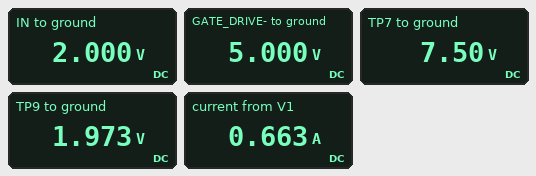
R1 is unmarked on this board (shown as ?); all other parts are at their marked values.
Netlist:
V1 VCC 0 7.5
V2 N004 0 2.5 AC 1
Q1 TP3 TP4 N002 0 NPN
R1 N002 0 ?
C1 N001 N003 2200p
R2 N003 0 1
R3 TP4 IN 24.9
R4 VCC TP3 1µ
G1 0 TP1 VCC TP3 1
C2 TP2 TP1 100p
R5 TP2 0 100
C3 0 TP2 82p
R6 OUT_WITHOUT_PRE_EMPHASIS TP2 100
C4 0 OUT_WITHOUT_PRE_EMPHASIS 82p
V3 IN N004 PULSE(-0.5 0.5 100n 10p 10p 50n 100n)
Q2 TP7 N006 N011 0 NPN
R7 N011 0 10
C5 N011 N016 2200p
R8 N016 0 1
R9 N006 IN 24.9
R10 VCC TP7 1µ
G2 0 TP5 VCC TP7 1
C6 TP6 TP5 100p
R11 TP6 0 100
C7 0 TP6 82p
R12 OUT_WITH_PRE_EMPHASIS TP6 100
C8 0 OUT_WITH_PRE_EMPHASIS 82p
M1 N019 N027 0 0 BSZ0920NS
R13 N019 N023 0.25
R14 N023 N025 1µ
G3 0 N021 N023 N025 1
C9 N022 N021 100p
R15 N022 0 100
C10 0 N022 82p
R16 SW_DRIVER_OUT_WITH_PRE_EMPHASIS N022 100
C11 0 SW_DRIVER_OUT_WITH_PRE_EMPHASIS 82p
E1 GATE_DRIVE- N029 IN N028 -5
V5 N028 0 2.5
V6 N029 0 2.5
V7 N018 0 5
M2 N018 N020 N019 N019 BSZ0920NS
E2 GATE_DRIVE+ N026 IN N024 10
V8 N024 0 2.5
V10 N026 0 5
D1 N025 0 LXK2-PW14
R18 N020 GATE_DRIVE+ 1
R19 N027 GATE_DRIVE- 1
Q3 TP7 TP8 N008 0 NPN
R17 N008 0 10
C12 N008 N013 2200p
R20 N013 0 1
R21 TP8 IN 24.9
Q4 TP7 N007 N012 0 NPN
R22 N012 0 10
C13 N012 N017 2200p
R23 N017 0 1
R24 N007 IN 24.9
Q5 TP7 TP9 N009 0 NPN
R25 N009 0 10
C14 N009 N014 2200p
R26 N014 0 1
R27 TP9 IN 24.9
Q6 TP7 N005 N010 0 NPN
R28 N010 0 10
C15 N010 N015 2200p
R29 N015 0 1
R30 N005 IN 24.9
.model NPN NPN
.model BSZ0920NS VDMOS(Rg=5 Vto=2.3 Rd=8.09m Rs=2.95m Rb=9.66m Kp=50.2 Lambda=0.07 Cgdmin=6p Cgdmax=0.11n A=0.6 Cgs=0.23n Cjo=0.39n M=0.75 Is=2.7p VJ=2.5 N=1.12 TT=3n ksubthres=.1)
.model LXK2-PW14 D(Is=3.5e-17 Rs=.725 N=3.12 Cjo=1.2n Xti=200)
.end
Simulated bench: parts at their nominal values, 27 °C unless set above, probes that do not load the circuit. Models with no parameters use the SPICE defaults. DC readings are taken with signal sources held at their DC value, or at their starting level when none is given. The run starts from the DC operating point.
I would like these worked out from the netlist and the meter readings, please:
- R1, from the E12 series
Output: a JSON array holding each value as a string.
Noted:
["8.2 Ω"]
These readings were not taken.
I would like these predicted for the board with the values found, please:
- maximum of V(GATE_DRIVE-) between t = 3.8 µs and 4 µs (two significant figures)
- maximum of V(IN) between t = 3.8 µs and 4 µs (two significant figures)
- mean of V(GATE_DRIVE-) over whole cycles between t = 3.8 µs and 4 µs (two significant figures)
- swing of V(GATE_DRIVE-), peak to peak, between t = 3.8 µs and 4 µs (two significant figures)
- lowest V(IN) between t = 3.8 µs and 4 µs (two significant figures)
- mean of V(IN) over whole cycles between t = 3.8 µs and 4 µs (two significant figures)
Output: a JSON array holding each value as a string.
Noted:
["5.0 V", "3.0 V", "2.5 V", "5.0 V", "2.0 V", "2.5 V"]
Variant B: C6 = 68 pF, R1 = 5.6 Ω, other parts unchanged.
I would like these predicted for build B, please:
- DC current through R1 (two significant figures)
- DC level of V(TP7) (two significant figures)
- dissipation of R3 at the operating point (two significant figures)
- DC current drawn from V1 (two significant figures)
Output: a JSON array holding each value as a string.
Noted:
["190 mA", "7.5 V", "85 µW", "720 mA"]
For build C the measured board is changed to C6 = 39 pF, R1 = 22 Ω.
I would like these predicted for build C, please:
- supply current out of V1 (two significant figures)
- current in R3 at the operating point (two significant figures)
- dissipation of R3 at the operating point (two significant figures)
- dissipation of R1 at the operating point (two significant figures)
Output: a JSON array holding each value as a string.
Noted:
["580 mA", "500 µA", "6.2 µW", "56 mW"]
